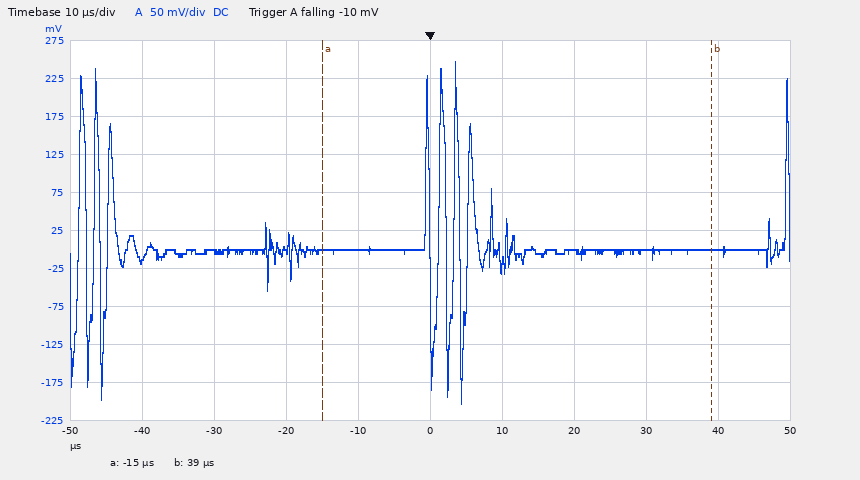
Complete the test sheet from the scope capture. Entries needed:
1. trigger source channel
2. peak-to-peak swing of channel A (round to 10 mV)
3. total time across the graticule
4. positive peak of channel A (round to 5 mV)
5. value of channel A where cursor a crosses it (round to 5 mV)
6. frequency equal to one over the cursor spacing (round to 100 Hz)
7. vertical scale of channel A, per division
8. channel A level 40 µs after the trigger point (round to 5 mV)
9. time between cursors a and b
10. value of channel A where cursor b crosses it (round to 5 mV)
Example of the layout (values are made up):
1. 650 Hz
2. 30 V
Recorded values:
1. channel A
2. 450 mV
3. 100 µs
4. 245 mV
5. 0 mV
6. 18.5 kHz
7. 50 mV
8. 0 mV
9. 54 µs
10. 0 mV
